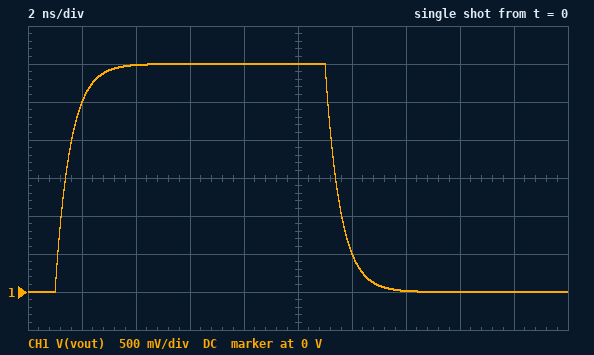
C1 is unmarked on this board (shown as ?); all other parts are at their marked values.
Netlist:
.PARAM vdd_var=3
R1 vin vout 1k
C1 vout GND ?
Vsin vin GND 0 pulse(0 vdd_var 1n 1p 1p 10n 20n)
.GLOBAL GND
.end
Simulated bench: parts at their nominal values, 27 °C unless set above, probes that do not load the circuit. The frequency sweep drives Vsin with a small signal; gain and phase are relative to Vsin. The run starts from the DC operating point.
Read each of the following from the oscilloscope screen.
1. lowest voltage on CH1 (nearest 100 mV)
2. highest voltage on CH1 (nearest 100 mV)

0 V
3.0 V
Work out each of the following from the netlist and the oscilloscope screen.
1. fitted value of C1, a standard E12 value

560 fF
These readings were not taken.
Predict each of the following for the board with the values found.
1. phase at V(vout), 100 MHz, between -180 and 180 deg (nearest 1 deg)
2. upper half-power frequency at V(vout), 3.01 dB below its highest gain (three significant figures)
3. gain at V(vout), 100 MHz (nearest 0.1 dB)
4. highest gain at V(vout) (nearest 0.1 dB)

-19 deg
284 MHz
-0.5 dB
0 dB
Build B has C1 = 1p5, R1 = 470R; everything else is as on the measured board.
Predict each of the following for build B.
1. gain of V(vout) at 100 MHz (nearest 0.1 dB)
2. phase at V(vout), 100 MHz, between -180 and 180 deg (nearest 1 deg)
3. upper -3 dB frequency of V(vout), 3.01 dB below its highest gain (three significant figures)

-0.8 dB
-24 deg
226 MHz
